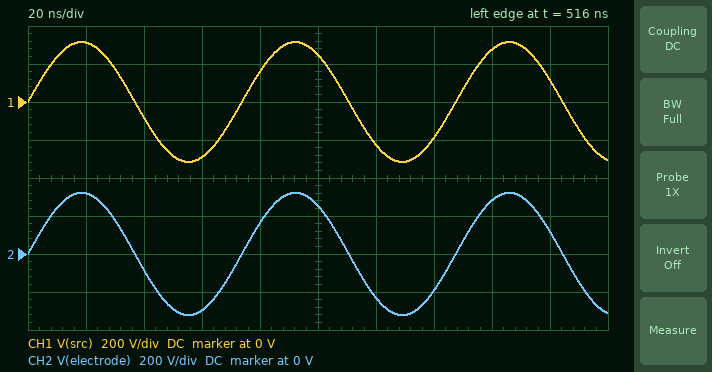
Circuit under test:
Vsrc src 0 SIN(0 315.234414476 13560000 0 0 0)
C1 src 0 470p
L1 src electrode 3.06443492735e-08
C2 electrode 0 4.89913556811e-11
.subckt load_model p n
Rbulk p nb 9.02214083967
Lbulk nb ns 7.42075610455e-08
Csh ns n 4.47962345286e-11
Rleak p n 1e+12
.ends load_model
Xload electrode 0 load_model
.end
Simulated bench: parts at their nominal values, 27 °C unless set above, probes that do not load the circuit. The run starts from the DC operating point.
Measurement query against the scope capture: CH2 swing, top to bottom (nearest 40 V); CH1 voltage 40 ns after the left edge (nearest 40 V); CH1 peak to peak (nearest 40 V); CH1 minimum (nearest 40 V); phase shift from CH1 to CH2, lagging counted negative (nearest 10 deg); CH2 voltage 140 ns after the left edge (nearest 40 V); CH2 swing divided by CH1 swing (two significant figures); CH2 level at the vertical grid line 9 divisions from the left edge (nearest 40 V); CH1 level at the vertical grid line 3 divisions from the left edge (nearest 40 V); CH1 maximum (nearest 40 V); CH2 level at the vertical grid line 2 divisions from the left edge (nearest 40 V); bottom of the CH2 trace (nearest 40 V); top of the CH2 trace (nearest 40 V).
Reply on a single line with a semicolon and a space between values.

640 V; -80 V; 640 V; -320 V; 0 deg; -200 V; 1.0; 120 V; -280 V; 320 V; -80 V; -320 V; 320 V
